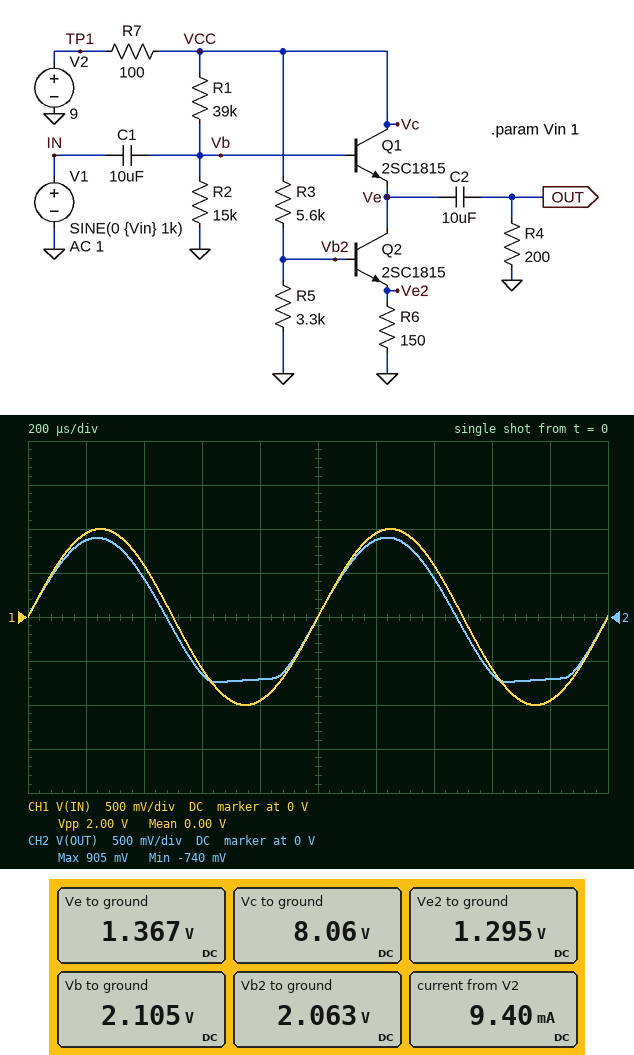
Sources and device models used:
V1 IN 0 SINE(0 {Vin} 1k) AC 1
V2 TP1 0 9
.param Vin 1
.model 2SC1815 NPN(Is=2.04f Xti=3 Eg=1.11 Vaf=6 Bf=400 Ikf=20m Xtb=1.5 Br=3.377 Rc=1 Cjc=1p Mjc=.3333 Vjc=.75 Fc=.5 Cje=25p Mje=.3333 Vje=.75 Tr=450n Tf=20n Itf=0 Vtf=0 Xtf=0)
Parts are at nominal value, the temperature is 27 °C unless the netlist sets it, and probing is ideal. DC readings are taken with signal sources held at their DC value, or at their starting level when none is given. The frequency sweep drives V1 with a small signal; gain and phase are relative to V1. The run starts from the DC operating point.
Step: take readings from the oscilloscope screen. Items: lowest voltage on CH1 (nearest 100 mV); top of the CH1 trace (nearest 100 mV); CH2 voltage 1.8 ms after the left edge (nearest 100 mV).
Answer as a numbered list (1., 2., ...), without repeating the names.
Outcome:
1. -1.0 V
2. 1.0 V
3. -700 mV
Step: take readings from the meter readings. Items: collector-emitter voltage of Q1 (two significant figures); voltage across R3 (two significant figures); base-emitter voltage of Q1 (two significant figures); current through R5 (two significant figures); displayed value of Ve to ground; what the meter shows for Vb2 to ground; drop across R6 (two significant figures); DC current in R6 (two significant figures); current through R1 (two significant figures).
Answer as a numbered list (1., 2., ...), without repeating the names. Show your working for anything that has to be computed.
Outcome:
1. 8.06 V - 1.367 V = 6.7 V
2. 8.06 V - 2.063 V = 6.0 V
3. 2.105 V - 1.367 V = 740 mV
4. (2.063 V) / 3.3 kΩ = 630 µA
5. 1.367 V
6. 2.063 V
7. 1.295 V = 1.3 V
8. (1.295 V) / 150 Ω = 8.6 mA
9. (8.06 V - 2.105 V) / 39 kΩ = 150 µA
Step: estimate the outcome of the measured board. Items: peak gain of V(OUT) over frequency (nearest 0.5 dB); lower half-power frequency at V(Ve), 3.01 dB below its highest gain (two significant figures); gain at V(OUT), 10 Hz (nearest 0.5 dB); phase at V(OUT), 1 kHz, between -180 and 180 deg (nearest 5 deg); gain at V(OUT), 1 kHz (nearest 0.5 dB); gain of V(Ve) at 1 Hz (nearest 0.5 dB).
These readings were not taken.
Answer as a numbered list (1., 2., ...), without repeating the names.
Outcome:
1. -0.5 dB
2. 1.9 Hz
3. -18.5 dB
4. 5 deg
5. -0.5 dB
6. -7.0 dB
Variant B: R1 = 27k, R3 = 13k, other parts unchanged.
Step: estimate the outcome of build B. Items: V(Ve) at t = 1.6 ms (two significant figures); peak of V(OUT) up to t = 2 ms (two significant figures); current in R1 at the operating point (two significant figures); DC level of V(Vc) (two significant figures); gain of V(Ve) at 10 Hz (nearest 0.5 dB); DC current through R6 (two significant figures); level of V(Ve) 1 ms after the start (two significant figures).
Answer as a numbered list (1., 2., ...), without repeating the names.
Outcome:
1. 1.6 V
2. 930 mV
3. 200 µA
4. 8.3 V
5. 0 dB
6. 6.0 mA
7. 2.2 V
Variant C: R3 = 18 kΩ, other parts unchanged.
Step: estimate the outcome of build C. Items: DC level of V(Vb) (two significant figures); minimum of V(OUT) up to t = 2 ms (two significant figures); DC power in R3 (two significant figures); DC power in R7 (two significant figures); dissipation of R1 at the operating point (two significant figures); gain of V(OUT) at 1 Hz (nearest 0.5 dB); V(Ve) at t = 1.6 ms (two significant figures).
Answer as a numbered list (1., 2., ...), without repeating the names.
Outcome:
1. 2.3 V
2. -810 mV
3. 2.9 mW
4. 1.9 mW
5. 1.0 mW
6. -43.0 dB
7. 1.1 V
